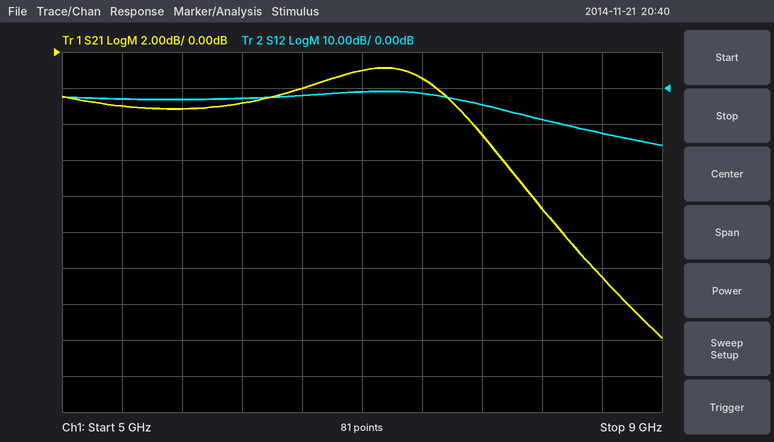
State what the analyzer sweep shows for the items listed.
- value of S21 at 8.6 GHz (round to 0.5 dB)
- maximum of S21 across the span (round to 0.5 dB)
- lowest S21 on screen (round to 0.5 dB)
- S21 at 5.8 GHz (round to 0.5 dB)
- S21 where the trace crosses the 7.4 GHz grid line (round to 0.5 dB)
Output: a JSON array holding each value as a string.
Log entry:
["-12.5 dB", "-1.0 dB", "-16.0 dB", "-3.0 dB", "-1.5 dB"]
